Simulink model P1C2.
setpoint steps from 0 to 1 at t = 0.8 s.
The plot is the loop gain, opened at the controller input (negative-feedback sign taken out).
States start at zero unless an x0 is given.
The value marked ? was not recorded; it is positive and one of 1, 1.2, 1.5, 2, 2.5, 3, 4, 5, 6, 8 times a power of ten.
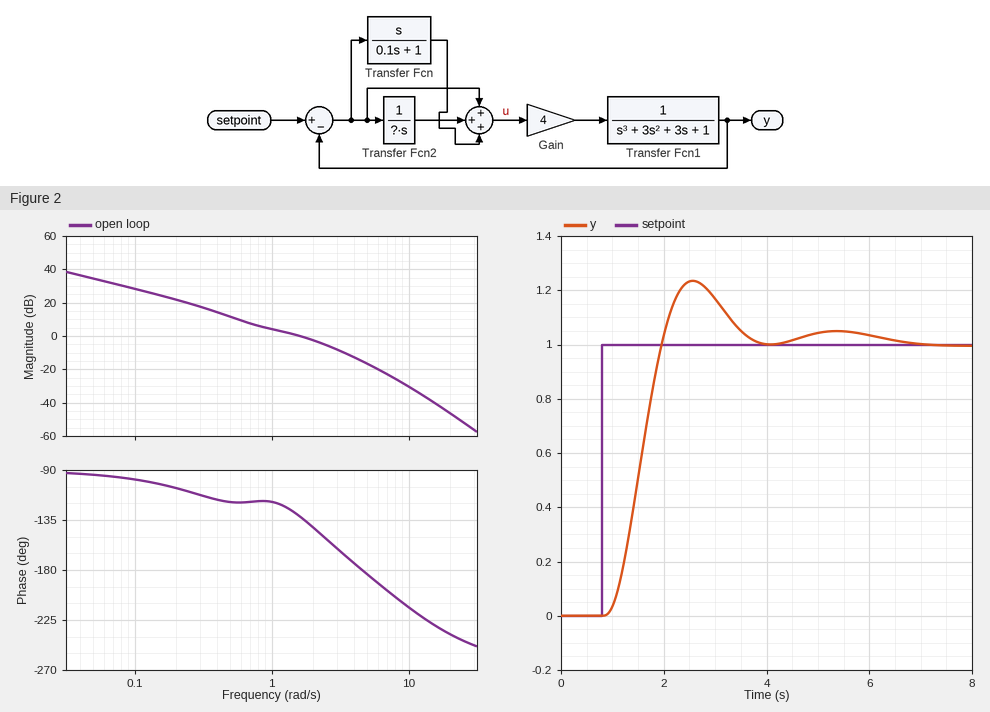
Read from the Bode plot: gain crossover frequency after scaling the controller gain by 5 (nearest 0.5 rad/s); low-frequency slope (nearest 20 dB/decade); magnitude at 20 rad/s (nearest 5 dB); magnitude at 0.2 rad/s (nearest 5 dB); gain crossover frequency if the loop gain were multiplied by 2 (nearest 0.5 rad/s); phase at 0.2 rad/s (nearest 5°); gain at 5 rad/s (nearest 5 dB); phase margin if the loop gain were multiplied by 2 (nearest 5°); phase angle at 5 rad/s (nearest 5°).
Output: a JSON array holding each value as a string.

["4.5 rad/s", "-20 dB/decade", "-45 dB", "20 dB", "2.5 rad/s", "-105°", "-15 dB", "25°", "-185°"]
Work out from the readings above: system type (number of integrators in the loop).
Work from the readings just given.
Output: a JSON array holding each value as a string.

["1"]
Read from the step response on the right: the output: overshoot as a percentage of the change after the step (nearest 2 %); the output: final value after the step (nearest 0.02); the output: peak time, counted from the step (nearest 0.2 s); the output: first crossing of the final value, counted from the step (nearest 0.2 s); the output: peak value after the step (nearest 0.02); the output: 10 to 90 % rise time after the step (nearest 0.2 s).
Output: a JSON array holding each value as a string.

["24 %", "1.00", "1.8 s", "1.2 s", "1.24", "0.8 s"]
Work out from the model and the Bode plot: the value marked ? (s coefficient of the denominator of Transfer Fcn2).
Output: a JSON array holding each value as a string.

["1.5"]
